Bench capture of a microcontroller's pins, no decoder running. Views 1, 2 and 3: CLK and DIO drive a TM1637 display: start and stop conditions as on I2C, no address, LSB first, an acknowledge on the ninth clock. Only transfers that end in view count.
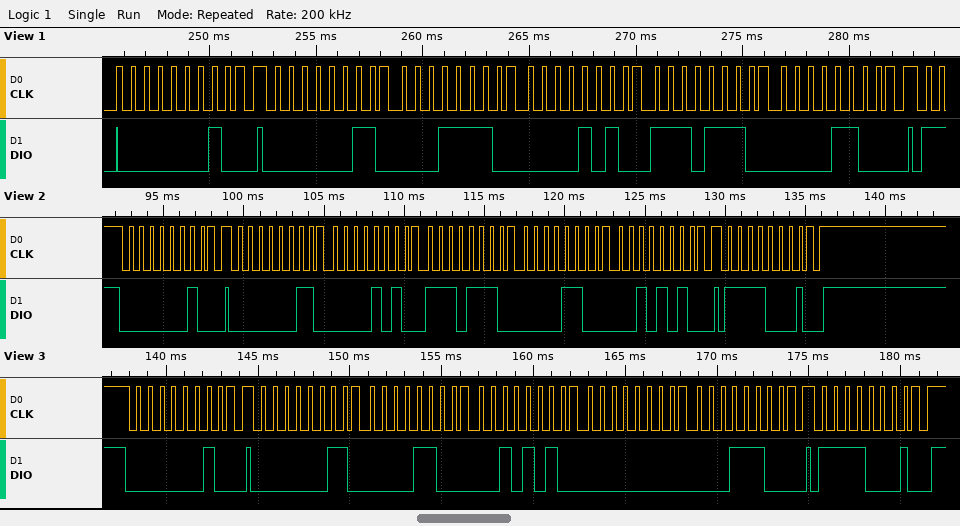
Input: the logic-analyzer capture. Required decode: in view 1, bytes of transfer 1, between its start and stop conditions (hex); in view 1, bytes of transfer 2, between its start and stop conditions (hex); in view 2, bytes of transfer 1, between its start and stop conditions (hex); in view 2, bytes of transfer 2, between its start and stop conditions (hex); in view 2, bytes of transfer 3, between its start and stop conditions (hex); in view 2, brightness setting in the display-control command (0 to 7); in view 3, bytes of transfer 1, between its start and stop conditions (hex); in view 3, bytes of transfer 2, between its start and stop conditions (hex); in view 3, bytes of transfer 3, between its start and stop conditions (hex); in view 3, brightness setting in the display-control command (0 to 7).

40
C0 78 50 77 30
40
C0 50 77 30 54
8F
7
40
C0 30 54 00 38
8F
7
